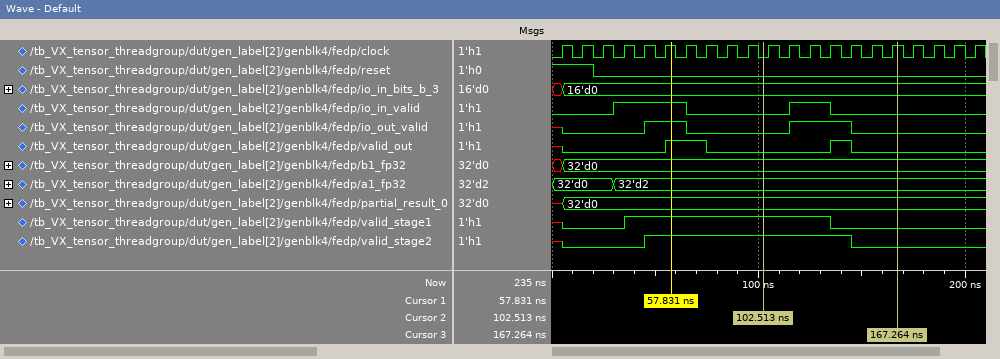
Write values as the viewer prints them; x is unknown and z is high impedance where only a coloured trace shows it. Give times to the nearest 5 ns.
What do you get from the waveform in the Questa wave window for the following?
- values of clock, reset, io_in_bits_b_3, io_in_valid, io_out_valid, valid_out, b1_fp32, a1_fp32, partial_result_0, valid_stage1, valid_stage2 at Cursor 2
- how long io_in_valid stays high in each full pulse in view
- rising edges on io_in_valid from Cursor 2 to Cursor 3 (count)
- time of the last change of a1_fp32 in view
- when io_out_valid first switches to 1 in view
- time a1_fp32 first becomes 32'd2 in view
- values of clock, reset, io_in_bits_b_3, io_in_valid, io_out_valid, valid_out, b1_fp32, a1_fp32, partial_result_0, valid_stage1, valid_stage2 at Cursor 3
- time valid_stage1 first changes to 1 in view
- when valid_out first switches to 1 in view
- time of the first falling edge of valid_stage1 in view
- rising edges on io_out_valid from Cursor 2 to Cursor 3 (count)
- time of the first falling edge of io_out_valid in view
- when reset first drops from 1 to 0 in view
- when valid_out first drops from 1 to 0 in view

clock=0, reset=0, io_in_bits_b_3=16'd0, io_in_valid=0, io_out_valid=0, valid_out=0, b1_fp32=32'd0, a1_fp32=32'd2, partial_result_0=32'd0, valid_stage1=1, valid_stage2=1
35 ns, 20 ns
1
30 ns
45 ns
30 ns
clock=1, reset=0, io_in_bits_b_3=16'd0, io_in_valid=0, io_out_valid=0, valid_out=0, b1_fp32=32'd0, a1_fp32=32'd2, partial_result_0=32'd0, valid_stage1=0, valid_stage2=0
35 ns
55 ns
135 ns
1
65 ns
20 ns
75 ns
